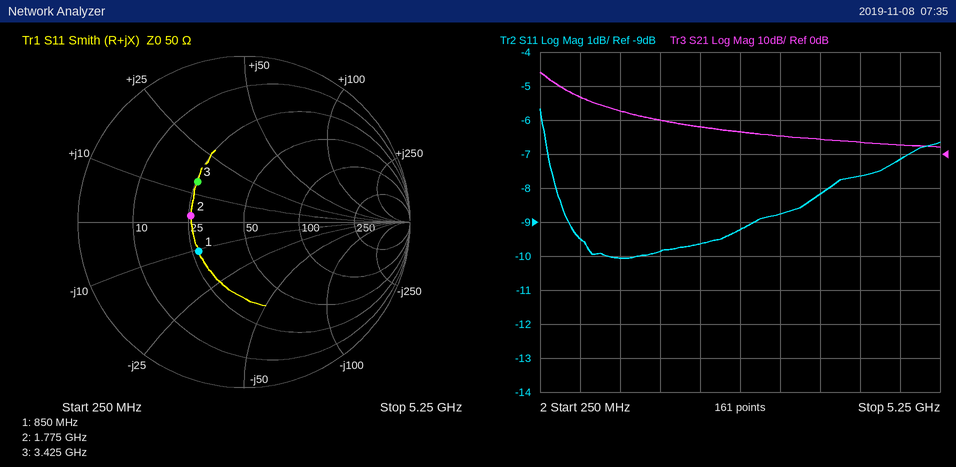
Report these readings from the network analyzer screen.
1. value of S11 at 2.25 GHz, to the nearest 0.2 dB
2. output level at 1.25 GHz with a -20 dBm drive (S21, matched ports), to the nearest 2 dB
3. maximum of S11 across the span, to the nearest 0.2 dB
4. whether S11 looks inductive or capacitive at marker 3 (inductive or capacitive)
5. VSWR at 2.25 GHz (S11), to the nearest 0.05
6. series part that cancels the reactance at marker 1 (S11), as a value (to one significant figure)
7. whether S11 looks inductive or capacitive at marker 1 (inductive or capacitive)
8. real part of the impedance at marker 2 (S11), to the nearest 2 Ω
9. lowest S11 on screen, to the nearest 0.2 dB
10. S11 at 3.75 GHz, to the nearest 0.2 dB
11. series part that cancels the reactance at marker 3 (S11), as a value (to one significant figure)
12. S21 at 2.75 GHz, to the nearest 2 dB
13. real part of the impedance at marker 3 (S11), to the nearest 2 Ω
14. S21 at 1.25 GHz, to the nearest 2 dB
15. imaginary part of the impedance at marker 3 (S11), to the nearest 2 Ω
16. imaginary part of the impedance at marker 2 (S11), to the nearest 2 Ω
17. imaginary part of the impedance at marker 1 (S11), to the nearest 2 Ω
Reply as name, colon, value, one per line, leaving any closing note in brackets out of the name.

value of S11 at 2.25 GHz, to the nearest 0.2 dB: -9.6 dB
output level at 1.25 GHz with a -20 dBm drive (S21, matched ports), to the nearest 2 dB: -8 dBm
maximum of S11 across the span, to the nearest 0.2 dB: -5.6 dB
whether S11 looks inductive or capacitive at marker 3: inductive
VSWR at 2.25 GHz (S11), to the nearest 0.05: 2.00
series part that cancels the reactance at marker 1 (S11), as a value: 2 nH
whether S11 looks inductive or capacitive at marker 1: capacitive
real part of the impedance at marker 2 (S11), to the nearest 2 Ω: 26 Ω
lowest S11 on screen, to the nearest 0.2 dB: -10.0 dB
S11 at 3.75 GHz, to the nearest 0.2 dB: -8.2 dB
series part that cancels the reactance at marker 3 (S11), as a value: 3 pF
S21 at 2.75 GHz, to the nearest 2 dB: 6 dB
real part of the impedance at marker 3 (S11), to the nearest 2 Ω: 26 Ω
S21 at 1.25 GHz, to the nearest 2 dB: 12 dB
imaginary part of the impedance at marker 3 (S11), to the nearest 2 Ω: +14 Ω
imaginary part of the impedance at marker 2 (S11), to the nearest 2 Ω: +2 Ω
imaginary part of the impedance at marker 1 (S11), to the nearest 2 Ω: -10 Ω
